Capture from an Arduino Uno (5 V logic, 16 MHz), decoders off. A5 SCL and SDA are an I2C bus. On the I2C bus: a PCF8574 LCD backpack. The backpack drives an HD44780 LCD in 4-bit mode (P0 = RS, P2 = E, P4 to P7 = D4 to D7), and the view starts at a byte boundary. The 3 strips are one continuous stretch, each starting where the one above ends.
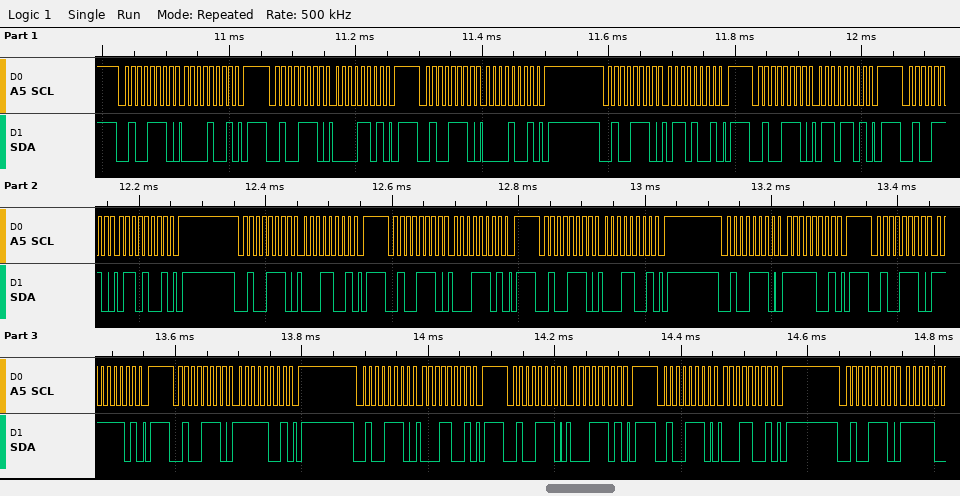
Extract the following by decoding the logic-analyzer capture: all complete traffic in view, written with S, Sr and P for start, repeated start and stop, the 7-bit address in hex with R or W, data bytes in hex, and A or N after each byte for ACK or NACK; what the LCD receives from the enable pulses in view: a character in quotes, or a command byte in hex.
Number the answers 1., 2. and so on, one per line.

1. S 27W A 09 A P S 27W A 0D A P S 27W A 09 A P S 27W A 69 A P S 27W A 6D A P S 27W A 69 A P S 27W A 19 A P S 27W A 1D A P S 27W A 19 A P S 27W A F9 A P S 27W A FD A P S 27W A F9 A P S 27W A 19 A P S 27W A 1D A P S 27W A 19 A P S 27W A
2. data 0x06 data 0x1F
